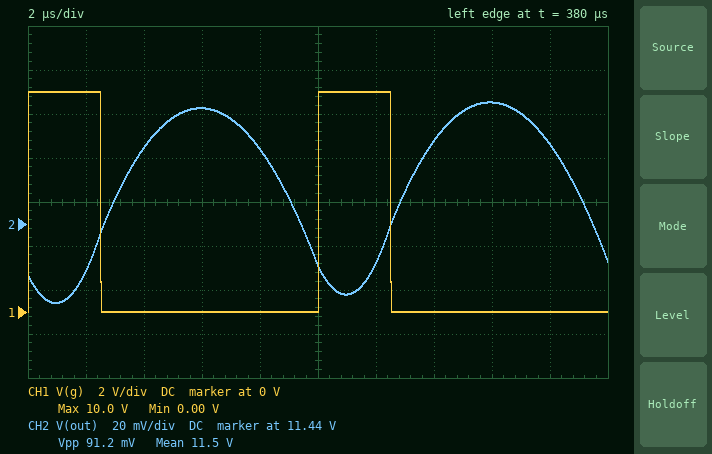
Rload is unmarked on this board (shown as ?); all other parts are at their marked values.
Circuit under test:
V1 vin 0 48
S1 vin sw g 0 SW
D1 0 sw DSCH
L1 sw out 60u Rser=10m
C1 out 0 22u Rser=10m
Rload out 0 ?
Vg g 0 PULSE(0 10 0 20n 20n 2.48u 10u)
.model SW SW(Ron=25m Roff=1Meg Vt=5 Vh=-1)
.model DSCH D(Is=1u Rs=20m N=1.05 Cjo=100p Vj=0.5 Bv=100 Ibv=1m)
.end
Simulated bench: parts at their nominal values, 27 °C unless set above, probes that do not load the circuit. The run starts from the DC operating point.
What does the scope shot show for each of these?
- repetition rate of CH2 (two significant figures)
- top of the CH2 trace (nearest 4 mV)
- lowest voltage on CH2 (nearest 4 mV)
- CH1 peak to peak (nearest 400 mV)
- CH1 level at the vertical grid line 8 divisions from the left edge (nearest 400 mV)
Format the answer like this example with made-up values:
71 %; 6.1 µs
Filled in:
100 kHz; 11.496 V; 11.404 V; 10.0 V; 0 V
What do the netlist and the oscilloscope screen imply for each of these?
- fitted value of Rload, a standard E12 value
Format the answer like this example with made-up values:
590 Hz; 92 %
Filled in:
1.5 Ω
